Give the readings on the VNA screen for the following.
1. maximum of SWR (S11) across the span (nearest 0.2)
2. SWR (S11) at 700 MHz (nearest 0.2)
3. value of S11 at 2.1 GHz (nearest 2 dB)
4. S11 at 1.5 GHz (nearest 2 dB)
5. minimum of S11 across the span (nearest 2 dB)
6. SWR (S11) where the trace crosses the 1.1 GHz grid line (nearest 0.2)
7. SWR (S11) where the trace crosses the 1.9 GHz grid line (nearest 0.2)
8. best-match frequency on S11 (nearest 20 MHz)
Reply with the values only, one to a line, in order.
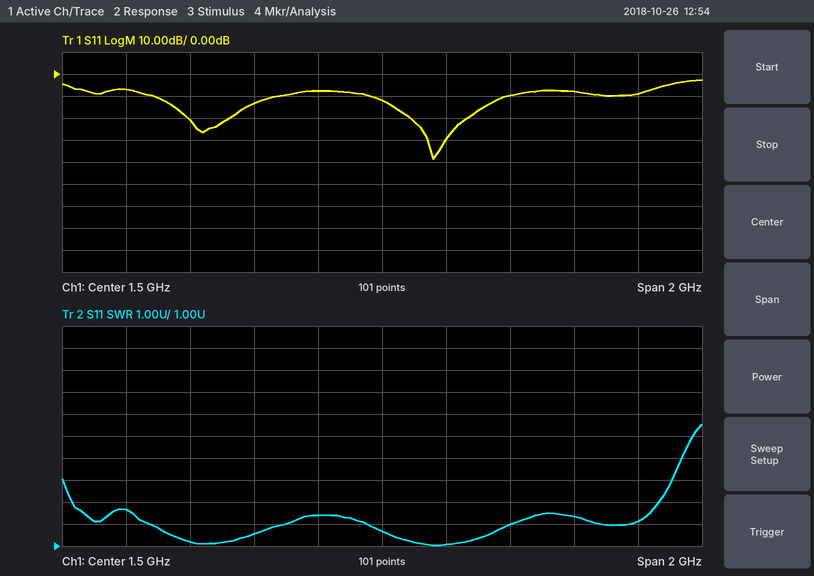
6.6
2.6
-8 dB
-12 dB
-38 dB
1.6
2.0
1.66 GHz
